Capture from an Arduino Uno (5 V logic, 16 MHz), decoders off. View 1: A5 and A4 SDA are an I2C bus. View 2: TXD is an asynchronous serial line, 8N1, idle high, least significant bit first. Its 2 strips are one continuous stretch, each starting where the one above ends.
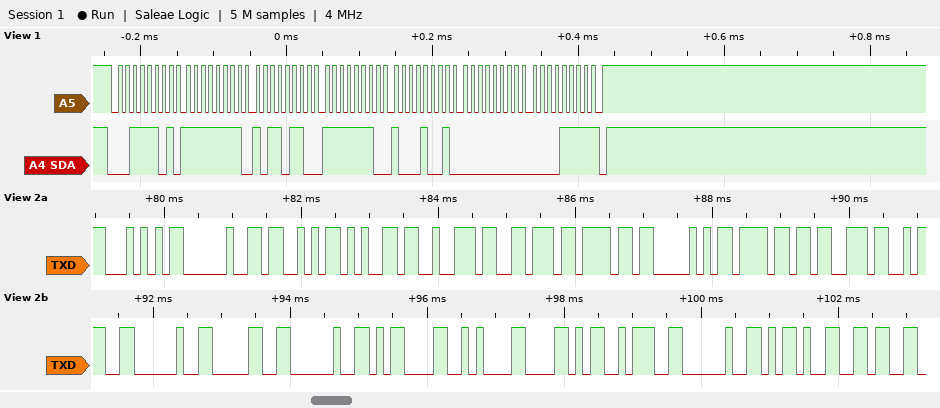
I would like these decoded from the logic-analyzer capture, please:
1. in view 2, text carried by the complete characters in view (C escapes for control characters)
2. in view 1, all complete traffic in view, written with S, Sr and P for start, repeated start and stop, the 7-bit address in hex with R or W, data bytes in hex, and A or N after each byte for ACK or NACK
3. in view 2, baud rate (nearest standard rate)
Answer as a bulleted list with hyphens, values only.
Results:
- "T ServoPos: 0 \r\nX: -6"
- S 1ER A FF A B6 A FE A 89 A 00 A 0F N P
- 9600 baud
